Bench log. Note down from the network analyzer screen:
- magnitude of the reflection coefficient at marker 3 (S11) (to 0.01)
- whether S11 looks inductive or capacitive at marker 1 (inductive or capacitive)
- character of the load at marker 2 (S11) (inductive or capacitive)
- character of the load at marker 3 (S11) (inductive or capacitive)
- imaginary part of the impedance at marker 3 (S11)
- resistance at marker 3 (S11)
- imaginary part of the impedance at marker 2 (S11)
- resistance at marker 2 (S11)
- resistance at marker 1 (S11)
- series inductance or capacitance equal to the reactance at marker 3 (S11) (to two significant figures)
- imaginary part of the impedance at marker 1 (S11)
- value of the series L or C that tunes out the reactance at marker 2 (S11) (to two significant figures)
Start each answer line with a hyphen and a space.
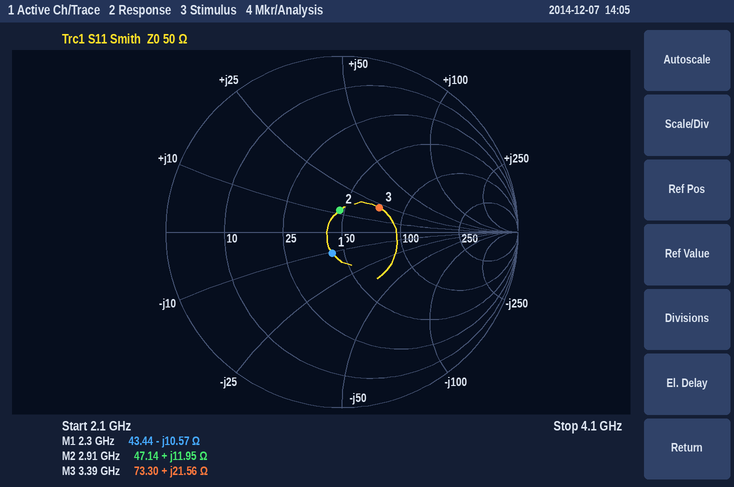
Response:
- 0.25
- capacitive
- inductive
- inductive
- +21.56 Ω
- 73.30 Ω
- +11.95 Ω
- 47.14 Ω
- 43.44 Ω
- 1.0 nH
- -10.57 Ω
- 4.6 pF
